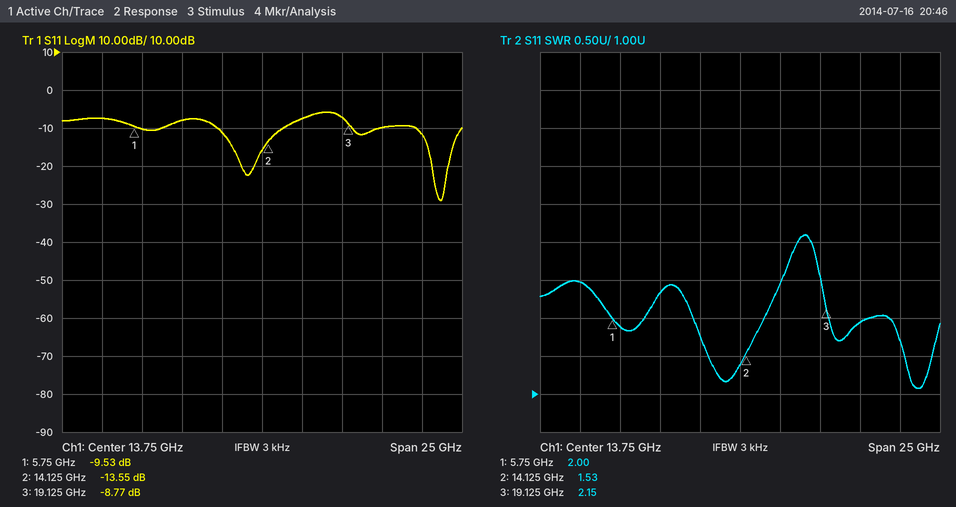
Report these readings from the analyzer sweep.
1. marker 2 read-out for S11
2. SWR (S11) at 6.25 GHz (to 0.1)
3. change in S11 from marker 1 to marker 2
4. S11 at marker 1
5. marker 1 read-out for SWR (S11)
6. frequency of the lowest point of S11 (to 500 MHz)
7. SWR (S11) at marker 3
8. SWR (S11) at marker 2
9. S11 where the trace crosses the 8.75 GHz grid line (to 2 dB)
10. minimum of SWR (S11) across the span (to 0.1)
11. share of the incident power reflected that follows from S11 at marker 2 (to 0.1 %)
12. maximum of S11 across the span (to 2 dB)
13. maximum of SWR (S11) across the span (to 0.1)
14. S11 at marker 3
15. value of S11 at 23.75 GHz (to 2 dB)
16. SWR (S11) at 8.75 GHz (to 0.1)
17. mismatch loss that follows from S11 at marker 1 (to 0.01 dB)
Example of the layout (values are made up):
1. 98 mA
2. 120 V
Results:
1. -13.55 dB
2. 1.9
3. -4.02 dB
4. -9.53 dB
5. 2.00
6. 25.0 GHz
7. 2.15
8. 1.53
9. -8 dB
10. 1.1
11. 4.4 %
12. -6 dB
13. 3.1
14. -8.77 dB
15. -12 dB
16. 2.3
17. 0.51 dB
